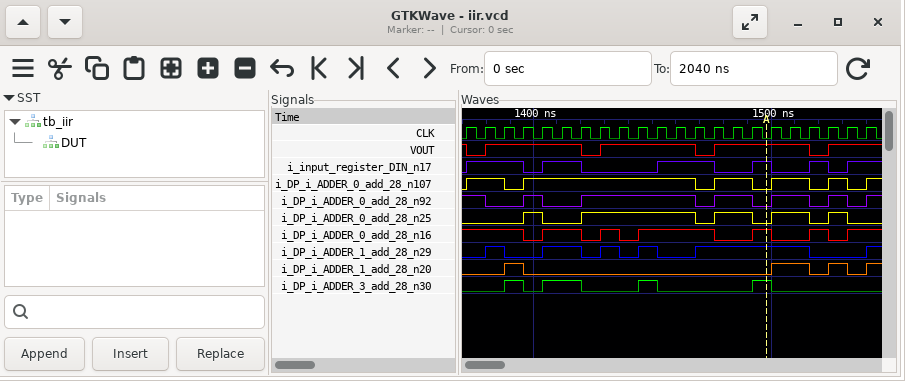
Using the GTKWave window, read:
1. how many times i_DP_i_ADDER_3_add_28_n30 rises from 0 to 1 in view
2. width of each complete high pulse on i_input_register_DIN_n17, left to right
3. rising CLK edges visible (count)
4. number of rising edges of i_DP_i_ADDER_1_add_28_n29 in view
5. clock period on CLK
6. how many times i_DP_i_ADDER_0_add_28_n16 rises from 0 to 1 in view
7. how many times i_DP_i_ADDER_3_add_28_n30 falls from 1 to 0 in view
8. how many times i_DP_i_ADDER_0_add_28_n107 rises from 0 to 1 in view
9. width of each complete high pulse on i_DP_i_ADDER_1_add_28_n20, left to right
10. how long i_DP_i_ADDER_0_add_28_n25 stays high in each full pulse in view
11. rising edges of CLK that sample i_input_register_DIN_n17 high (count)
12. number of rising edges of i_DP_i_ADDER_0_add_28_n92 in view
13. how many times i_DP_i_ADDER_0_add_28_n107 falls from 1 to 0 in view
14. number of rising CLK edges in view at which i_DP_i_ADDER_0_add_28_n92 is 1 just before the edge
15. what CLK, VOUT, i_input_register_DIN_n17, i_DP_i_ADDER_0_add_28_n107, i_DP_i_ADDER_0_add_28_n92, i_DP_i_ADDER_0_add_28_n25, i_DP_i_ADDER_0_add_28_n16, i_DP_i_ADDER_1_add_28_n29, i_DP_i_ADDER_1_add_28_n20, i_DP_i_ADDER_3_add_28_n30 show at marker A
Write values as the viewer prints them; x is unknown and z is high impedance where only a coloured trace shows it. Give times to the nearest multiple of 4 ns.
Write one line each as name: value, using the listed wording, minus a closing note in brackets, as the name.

how many times i_DP_i_ADDER_3_add_28_n30 rises from 0 to 1 in view: 4
width of each complete high pulse on i_input_register_DIN_n17, left to right: 24 ns, 16 ns, 24 ns, 8 ns, 8 ns
rising CLK edges visible: 22
number of rising edges of i_DP_i_ADDER_1_add_28_n29 in view: 6
clock period on CLK: 8 ns
how many times i_DP_i_ADDER_0_add_28_n16 rises from 0 to 1 in view: 6
how many times i_DP_i_ADDER_3_add_28_n30 falls from 1 to 0 in view: 4
how many times i_DP_i_ADDER_0_add_28_n107 rises from 0 to 1 in view: 6
width of each complete high pulse on i_DP_i_ADDER_1_add_28_n20, left to right: 8 ns, 16 ns, 8 ns
how long i_DP_i_ADDER_0_add_28_n25 stays high in each full pulse in view: 8 ns, 48 ns, 16 ns, 16 ns, 8 ns
rising edges of CLK that sample i_input_register_DIN_n17 high: 11
number of rising edges of i_DP_i_ADDER_0_add_28_n92 in view: 6
how many times i_DP_i_ADDER_0_add_28_n107 falls from 1 to 0 in view: 5
number of rising CLK edges in view at which i_DP_i_ADDER_0_add_28_n92 is 1 just before the edge: 14
what CLK, VOUT, i_input_register_DIN_n17, i_DP_i_ADDER_0_add_28_n107, i_DP_i_ADDER_0_add_28_n92, i_DP_i_ADDER_0_add_28_n25, i_DP_i_ADDER_0_add_28_n16, i_DP_i_ADDER_1_add_28_n29, i_DP_i_ADDER_1_add_28_n20, i_DP_i_ADDER_3_add_28_n30 show at marker A: CLK=0, VOUT=1, i_input_register_DIN_n17=1, i_DP_i_ADDER_0_add_28_n107=0, i_DP_i_ADDER_0_add_28_n92=0, i_DP_i_ADDER_0_add_28_n25=0, i_DP_i_ADDER_0_add_28_n16=1, i_DP_i_ADDER_1_add_28_n29=1, i_DP_i_ADDER_1_add_28_n20=0, i_DP_i_ADDER_3_add_28_n30=1
